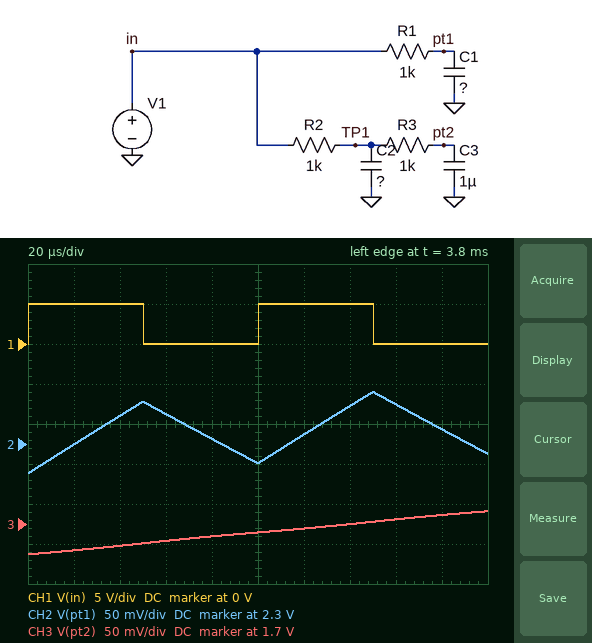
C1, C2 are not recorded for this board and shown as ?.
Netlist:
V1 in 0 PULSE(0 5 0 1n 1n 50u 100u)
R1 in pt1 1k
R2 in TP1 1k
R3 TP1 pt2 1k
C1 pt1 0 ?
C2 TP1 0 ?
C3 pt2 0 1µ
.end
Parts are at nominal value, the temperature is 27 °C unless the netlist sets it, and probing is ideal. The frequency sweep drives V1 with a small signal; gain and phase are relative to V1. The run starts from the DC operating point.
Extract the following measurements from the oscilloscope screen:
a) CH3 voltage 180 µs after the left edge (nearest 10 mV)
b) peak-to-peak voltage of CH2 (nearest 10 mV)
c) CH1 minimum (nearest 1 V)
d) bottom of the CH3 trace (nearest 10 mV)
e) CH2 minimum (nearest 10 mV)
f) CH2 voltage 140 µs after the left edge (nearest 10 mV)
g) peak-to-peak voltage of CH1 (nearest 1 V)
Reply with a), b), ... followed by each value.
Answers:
a) 1.71 V
b) 100 mV
c) 0 V
d) 1.66 V
e) 2.26 V
f) 2.35 V
g) 5 V
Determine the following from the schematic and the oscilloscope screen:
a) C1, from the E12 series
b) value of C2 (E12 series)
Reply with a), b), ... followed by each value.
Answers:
a) 1.5 µF
b) 1.5 µF
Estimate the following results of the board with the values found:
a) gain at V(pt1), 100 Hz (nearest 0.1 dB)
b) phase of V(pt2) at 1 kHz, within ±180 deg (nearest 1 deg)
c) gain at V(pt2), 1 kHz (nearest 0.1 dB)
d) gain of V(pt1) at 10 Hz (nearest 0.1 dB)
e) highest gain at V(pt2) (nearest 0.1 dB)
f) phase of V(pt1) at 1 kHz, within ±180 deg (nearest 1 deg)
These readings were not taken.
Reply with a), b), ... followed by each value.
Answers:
a) -2.8 dB
b) -159 deg
c) -35.9 dB
d) 0 dB
e) 0 dB
f) -84 deg
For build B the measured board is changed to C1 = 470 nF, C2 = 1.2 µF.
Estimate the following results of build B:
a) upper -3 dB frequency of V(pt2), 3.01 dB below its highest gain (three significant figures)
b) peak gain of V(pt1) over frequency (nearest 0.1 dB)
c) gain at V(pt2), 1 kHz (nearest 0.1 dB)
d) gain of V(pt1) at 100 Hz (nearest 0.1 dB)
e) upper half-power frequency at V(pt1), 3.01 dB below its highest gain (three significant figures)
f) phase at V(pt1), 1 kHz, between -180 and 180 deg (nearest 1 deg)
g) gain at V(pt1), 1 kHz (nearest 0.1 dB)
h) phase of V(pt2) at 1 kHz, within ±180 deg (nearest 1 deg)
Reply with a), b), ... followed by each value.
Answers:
a) 56.2 Hz
b) 0 dB
c) -34.1 dB
d) -0.4 dB
e) 339 Hz
f) -71 deg
g) -9.9 dB
h) -157 deg
